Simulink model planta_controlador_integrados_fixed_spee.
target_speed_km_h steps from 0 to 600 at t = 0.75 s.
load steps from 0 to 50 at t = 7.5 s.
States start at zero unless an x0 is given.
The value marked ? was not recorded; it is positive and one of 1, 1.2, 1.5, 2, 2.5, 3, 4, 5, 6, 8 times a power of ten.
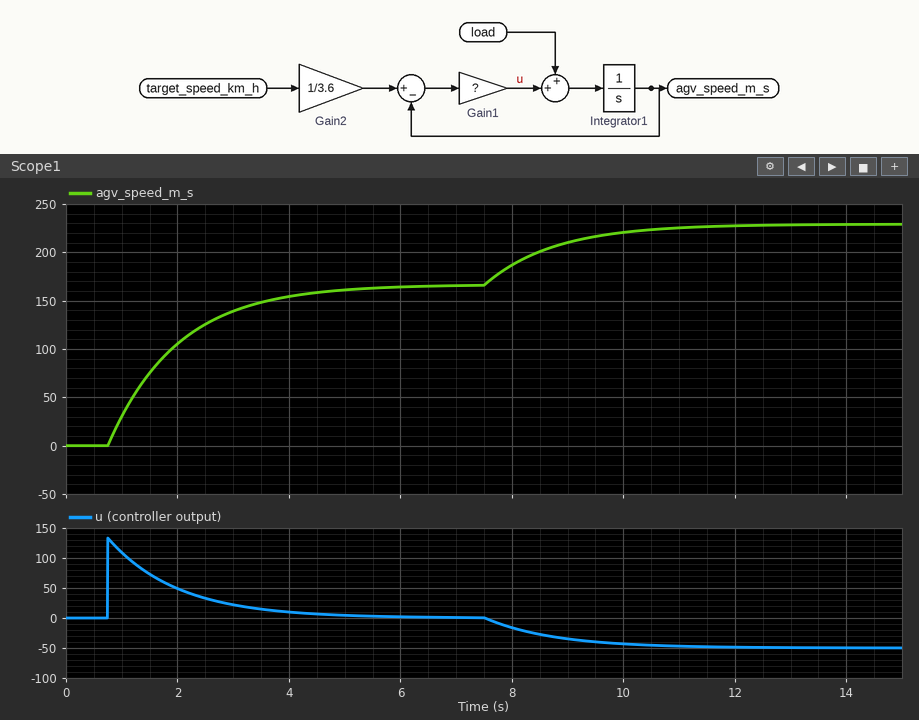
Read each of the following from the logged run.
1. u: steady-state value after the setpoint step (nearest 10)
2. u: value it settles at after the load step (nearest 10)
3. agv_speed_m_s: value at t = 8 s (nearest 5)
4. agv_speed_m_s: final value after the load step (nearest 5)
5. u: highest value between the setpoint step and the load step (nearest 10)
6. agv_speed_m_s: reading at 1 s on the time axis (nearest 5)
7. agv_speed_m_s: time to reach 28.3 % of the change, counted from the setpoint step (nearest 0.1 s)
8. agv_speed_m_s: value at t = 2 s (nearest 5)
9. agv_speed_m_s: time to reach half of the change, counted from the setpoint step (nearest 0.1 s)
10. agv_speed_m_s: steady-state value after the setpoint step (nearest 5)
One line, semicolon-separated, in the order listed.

0; -50; 185; 230; 130; 30; 0.4 s; 105; 0.9 s; 165
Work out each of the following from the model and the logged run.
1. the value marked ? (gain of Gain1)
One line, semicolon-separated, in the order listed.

0.8
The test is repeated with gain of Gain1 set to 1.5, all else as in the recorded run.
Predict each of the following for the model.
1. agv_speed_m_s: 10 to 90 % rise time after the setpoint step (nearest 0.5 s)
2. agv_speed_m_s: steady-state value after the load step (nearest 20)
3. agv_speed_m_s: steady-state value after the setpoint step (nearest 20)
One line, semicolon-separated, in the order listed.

1.5 s; 200; 160
